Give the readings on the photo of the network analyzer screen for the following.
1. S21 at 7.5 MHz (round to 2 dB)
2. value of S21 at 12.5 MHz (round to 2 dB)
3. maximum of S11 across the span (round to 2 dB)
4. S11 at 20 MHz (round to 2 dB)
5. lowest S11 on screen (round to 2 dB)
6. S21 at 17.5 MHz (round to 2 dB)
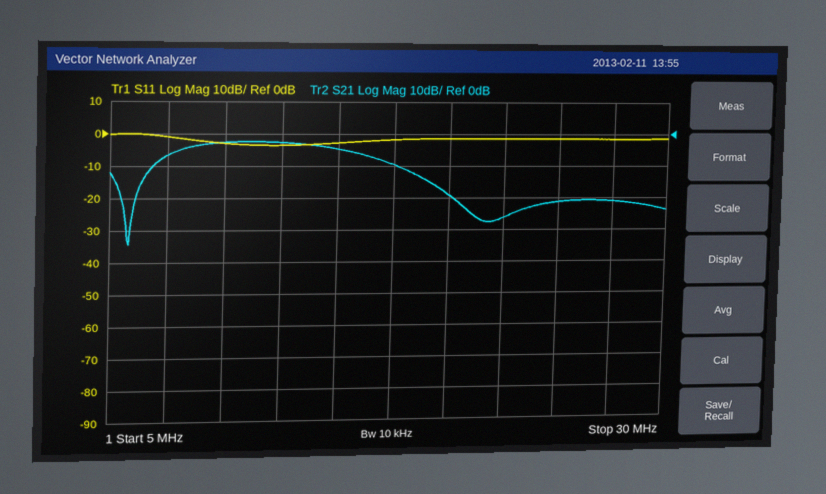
-6 dB
-2 dB
0 dB
-2 dB
-4 dB
-10 dB
